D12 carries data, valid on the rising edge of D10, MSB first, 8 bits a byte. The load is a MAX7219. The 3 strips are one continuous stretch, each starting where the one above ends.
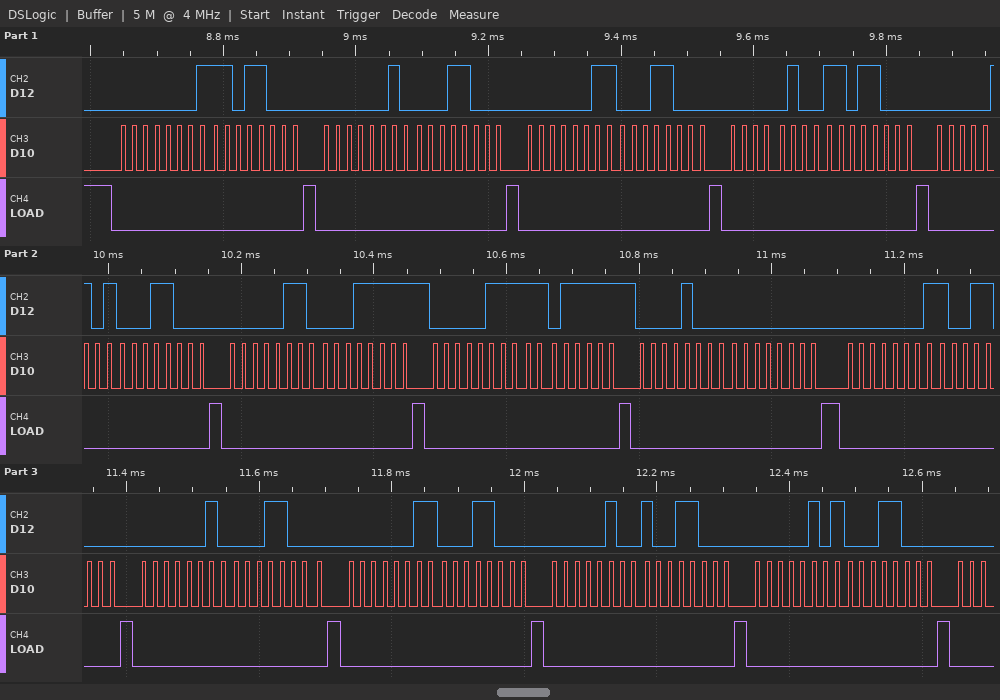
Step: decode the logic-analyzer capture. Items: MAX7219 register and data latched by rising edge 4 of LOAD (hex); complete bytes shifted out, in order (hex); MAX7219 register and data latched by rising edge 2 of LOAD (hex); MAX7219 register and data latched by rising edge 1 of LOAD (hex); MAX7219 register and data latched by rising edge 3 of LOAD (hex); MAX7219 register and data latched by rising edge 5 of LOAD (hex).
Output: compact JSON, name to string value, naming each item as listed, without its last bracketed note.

{"MAX7219 register and data latched by rising edge 4 of LOAD": "register 0x4, data 0xD8", "complete bytes shifted out, in order": "0x01 0xD8 0x02 0x18 0x03 0x18 0x04 0xD8 0x05 0x18 0x06 0x1F 0x07 0xDF 0x08 0x00 0x01 0x98 0x02 0x18 0x03 0x18 0x04 0x98 0x05 0x18", "MAX7219 register and data latched by rising edge 2 of LOAD": "register 0x2, data 0x18", "MAX7219 register and data latched by rising edge 1 of LOAD": "register 0x1, data 0xD8", "MAX7219 register and data latched by rising edge 3 of LOAD": "register 0x3, data 0x18", "MAX7219 register and data latched by rising edge 5 of LOAD": "register 0x5, data 0x18"}
